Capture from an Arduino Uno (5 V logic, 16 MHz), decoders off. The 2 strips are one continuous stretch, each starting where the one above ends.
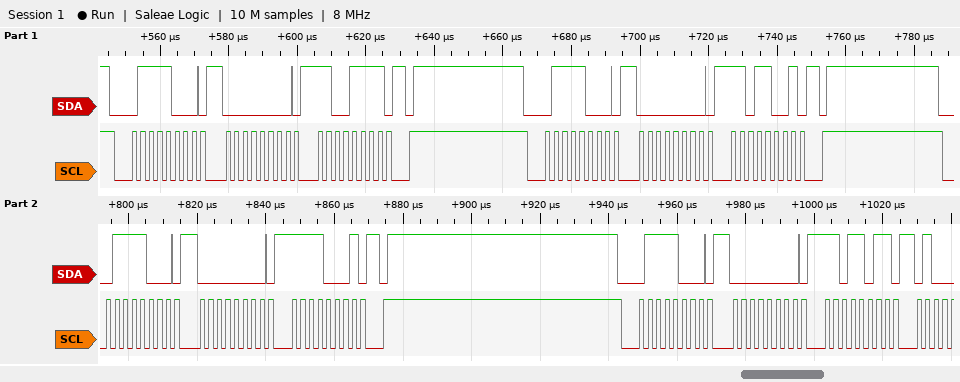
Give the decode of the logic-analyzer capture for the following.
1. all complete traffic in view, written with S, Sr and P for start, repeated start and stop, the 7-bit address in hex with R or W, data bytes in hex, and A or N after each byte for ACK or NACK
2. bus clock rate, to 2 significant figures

S 3CW A 00 A CF A P S 3CW A 00 A D9 A P S 3CW A 00 A F1 A P S 3CW A 00 A DB A
400 kHz
